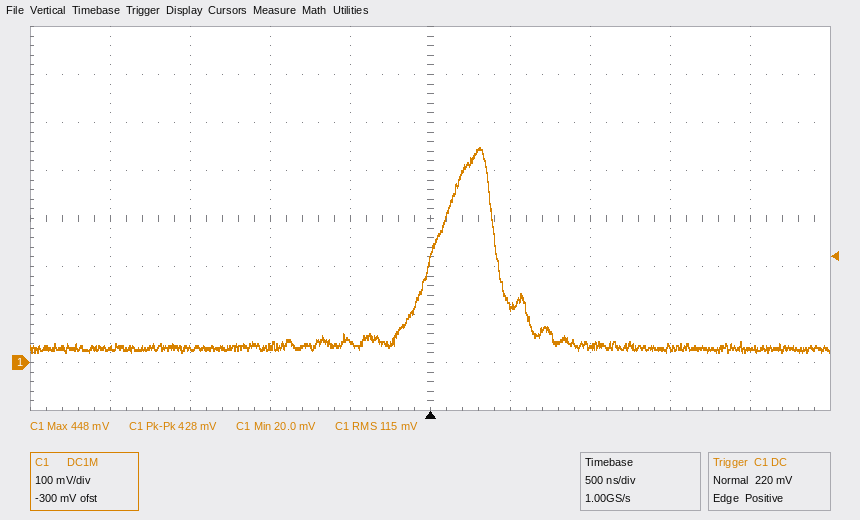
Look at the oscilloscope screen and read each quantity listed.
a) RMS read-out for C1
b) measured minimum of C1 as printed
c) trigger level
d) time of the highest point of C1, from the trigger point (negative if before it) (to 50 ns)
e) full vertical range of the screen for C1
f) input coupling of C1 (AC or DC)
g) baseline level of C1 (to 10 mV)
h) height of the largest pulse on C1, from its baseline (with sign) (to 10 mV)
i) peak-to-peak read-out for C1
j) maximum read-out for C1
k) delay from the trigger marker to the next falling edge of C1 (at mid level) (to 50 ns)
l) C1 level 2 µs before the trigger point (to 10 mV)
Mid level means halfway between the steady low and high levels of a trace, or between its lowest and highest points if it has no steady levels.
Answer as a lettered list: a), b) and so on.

a) 115 mV
b) 20.0 mV
c) 220 mV
d) +300 ns
e) 800 mV
f) DC
g) 30 mV
h) +420 mV
i) 428 mV
j) 448 mV
k) 400 ns
l) 30 mV
